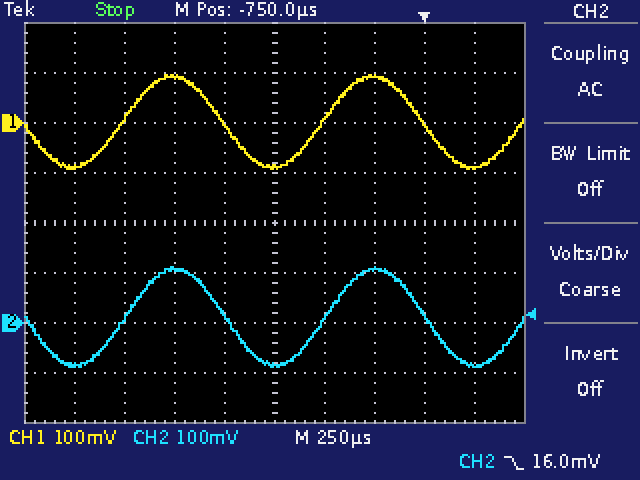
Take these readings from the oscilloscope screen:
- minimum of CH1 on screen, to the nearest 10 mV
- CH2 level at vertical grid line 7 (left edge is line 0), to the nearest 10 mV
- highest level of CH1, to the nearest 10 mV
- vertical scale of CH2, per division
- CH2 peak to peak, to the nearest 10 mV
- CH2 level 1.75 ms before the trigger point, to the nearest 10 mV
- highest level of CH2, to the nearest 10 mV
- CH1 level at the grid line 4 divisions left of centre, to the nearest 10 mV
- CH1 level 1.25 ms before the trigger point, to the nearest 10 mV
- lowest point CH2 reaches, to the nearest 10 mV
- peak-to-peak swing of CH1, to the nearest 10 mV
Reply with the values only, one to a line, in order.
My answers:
-90 mV
110 mV
100 mV
100 mV
200 mV
-80 mV
110 mV
-90 mV
90 mV
-90 mV
190 mV
